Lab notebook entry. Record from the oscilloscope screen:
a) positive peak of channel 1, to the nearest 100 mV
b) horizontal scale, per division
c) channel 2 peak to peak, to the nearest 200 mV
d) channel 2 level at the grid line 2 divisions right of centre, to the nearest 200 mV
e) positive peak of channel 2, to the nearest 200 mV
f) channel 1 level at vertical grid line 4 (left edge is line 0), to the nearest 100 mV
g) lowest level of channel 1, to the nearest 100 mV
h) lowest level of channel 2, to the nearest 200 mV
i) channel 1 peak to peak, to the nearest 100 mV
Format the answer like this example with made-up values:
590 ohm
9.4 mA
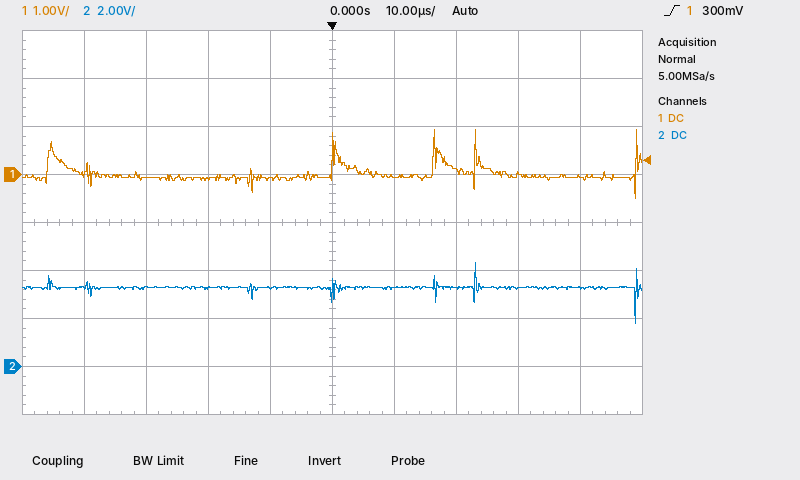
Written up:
900 mV
10 µs
2.6 V
3.2 V
4.4 V
-100 mV
-500 mV
1.8 V
1.4 V
